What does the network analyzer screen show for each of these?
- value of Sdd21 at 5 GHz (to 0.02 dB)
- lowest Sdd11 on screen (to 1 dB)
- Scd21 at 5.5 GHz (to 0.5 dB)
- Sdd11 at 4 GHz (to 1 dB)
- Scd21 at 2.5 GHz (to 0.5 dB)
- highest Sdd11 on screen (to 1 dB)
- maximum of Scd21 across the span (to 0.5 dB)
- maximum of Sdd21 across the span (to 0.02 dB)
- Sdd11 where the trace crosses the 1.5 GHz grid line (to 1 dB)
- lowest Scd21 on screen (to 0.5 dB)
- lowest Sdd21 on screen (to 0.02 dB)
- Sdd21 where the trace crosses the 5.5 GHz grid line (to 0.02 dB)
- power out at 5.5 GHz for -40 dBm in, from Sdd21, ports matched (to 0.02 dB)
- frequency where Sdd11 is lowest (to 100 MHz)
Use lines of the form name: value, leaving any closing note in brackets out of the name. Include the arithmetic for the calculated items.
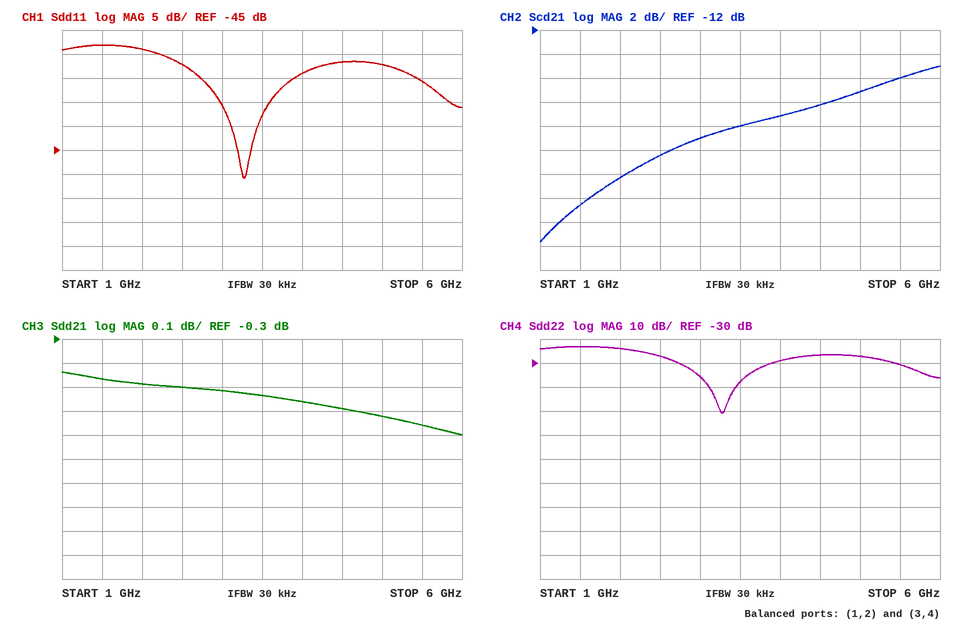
value of Sdd21 at 5 GHz: -0.62 dB
lowest Sdd11 on screen: -51 dB
Scd21 at 5.5 GHz: -16.0 dB
Sdd11 at 4 GHz: -29 dB
Scd21 at 2.5 GHz: -22.5 dB
highest Sdd11 on screen: -23 dB
maximum of Scd21 across the span: -15.0 dB
maximum of Sdd21 across the span: -0.44 dB
Sdd11 where the trace crosses the 1.5 GHz grid line: -23 dB
lowest Scd21 on screen: -29.5 dB
lowest Sdd21 on screen: -0.70 dB
Sdd21 where the trace crosses the 5.5 GHz grid line: -0.66 dB
power out at 5.5 GHz for -40 dBm in, from Sdd21, ports matched: -40 dBm + (-0.66 dB) = -40.66 dBm
frequency where Sdd11 is lowest: 3.3 GHz
